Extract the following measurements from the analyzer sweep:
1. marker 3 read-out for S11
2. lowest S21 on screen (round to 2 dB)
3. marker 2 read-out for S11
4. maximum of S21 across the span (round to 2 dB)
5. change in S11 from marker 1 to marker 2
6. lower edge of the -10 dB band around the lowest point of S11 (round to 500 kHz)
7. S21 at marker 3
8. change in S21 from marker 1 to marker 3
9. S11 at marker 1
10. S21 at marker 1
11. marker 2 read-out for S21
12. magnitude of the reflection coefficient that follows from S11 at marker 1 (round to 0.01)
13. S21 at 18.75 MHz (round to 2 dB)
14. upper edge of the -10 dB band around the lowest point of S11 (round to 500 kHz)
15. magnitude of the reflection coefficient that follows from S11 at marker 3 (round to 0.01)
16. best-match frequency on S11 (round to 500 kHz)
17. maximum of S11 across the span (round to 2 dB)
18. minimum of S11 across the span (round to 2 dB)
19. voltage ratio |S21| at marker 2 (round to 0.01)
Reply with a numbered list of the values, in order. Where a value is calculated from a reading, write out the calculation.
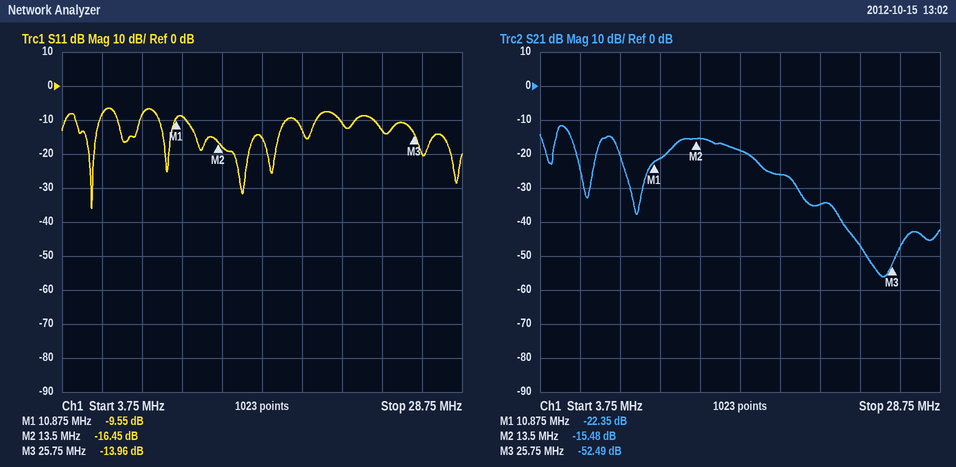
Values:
1. -13.96 dB
2. -56 dB
3. -16.45 dB
4. -12 dB
5. -16.45 − (-9.55) = -6.90 dB
6. 4.5 MHz
7. -52.49 dB
8. -52.49 − (-22.35) = -30.14 dB
9. -9.55 dB
10. -22.35 dB
11. -15.48 dB
12. 10^(-9.55/20) ≈ 0.33
13. -26 dB
14. 6.0 MHz
15. 10^(-13.96/20) ≈ 0.20
16. 5.5 MHz
17. -6 dB
18. -36 dB
19. 10^(-15.48/20) ≈ 0.17
